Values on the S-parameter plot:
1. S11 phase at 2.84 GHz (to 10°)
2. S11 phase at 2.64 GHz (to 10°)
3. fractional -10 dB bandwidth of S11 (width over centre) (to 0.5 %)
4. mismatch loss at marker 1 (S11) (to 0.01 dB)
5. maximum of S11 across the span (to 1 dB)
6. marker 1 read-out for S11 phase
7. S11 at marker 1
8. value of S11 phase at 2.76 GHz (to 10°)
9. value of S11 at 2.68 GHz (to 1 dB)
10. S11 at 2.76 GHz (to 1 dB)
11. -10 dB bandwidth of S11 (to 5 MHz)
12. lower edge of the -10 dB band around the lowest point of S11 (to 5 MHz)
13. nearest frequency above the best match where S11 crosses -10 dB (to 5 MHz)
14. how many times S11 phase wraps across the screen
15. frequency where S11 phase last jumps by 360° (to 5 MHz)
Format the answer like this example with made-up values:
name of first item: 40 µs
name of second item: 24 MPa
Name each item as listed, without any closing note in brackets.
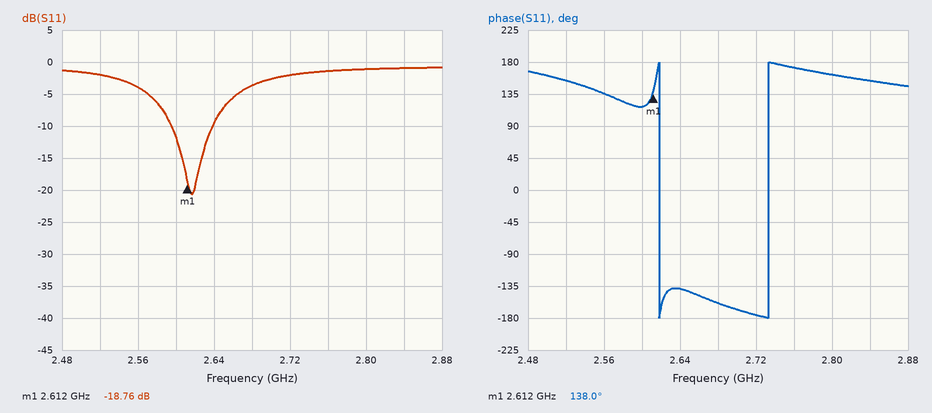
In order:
S11 phase at 2.84 GHz: 150°
S11 phase at 2.64 GHz: -140°
fractional -10 dB bandwidth of S11 (width over centre): 1.5 %
mismatch loss at marker 1 (S11): 0.06 dB
maximum of S11 across the span: -1 dB
marker 1 read-out for S11 phase: 138.0°
S11 at marker 1: -18.76 dB
value of S11 phase at 2.76 GHz: 170°
value of S11 at 2.68 GHz: -4 dB
S11 at 2.76 GHz: -1 dB
-10 dB bandwidth of S11: 45 MHz
lower edge of the -10 dB band around the lowest point of S11: 2.595 GHz
nearest frequency above the best match where S11 crosses -10 dB: 2.640 GHz
how many times S11 phase wraps across the screen: 2
frequency where S11 phase last jumps by 360°: 2.735 GHz
